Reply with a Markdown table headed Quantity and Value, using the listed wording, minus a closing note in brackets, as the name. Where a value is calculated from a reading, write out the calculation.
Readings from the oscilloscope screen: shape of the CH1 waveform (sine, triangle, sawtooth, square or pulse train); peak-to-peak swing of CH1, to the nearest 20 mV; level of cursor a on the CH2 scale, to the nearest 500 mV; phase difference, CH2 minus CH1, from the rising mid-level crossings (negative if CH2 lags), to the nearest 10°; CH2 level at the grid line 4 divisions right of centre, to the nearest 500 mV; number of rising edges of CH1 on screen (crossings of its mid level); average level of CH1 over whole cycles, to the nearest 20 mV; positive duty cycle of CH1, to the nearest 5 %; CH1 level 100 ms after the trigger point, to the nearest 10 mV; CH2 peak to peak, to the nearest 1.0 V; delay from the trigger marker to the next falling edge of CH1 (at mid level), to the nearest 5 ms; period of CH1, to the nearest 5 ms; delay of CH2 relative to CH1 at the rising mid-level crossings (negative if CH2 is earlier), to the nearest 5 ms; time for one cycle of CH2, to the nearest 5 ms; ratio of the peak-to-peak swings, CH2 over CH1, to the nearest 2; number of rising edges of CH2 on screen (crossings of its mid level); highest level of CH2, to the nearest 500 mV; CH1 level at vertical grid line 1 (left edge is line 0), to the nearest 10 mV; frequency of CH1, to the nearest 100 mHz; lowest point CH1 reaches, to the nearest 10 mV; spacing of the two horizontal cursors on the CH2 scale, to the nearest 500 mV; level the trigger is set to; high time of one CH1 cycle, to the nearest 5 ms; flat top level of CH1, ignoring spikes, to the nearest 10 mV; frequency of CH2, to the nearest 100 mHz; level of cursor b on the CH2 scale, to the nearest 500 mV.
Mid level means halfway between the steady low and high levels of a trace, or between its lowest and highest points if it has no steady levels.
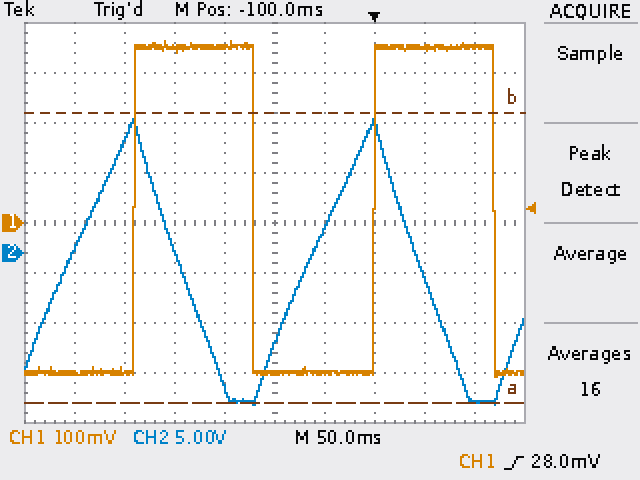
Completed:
| Quantity | Value |
|---|---|
| shape of the CH1 waveform | square |
| peak-to-peak swing of CH1, to the nearest 20 mV | 680 mV |
| level of cursor a on the CH2 scale, to the nearest 500 mV | -15.0 V |
| phase difference, CH2 minus CH1, from the rising mid-level crossings (negative if CH2 lags), to the nearest 10° | −360° × (-65 ms) / 240 ms ≈ +97.5°, so +100° to the nearest 10° |
| CH2 level at the grid line 4 divisions right of centre, to the nearest 500 mV | -15.0 V |
| number of rising edges of CH1 on screen | 2 |
| average level of CH1 over whole cycles, to the nearest 20 mV | -310 mV + 0.5 × (350 mV − (-310 mV)) ≈ 20 mV |
| positive duty cycle of CH1, to the nearest 5 % | 120 ms / 240 ms ≈ 50 % |
| CH1 level 100 ms after the trigger point, to the nearest 10 mV | 350 mV |
| CH2 peak to peak, to the nearest 1.0 V | 29.0 V |
| delay from the trigger marker to the next falling edge of CH1 (at mid level), to the nearest 5 ms | 120 ms |
| period of CH1, to the nearest 5 ms | 240 ms |
| delay of CH2 relative to CH1 at the rising mid-level crossings (negative if CH2 is earlier), to the nearest 5 ms | -65 ms |
| time for one cycle of CH2, to the nearest 5 ms | 240 ms |
| ratio of the peak-to-peak swings, CH2 over CH1, to the nearest 2 | 29.0 V / 680 mV ≈ 42.6, so 42 to the nearest 2 |
| number of rising edges of CH2 on screen | 2 |
| highest level of CH2, to the nearest 500 mV | 13.5 V |
| CH1 level at vertical grid line 1 (left edge is line 0), to the nearest 10 mV | -300 mV |
| frequency of CH1, to the nearest 100 mHz | 1 / 240 ms ≈ 4.2 Hz |
| lowest point CH1 reaches, to the nearest 10 mV | -310 mV |
| spacing of the two horizontal cursors on the CH2 scale, to the nearest 500 mV | 29.0 V |
| level the trigger is set to | 28.0 mV |
| high time of one CH1 cycle, to the nearest 5 ms | 120 ms |
| flat top level of CH1, ignoring spikes, to the nearest 10 mV | 350 mV |
| frequency of CH2, to the nearest 100 mHz | 1 / 240 ms ≈ 4.2 Hz |
| level of cursor b on the CH2 scale, to the nearest 500 mV | 14.0 V |
